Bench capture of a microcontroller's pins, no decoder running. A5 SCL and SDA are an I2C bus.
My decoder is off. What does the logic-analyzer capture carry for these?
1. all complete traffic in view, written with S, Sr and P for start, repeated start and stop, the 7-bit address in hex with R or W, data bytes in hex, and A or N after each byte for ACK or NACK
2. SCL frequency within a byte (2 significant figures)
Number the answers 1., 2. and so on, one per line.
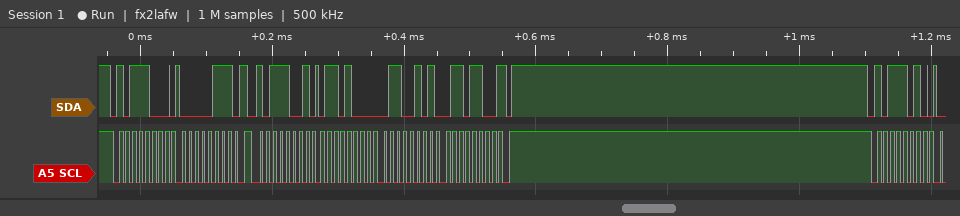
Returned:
1. S 5CW A 07 A Sr 5CR A 68 A 65 A 6C N P S 5DW A
2. 100 kHz
